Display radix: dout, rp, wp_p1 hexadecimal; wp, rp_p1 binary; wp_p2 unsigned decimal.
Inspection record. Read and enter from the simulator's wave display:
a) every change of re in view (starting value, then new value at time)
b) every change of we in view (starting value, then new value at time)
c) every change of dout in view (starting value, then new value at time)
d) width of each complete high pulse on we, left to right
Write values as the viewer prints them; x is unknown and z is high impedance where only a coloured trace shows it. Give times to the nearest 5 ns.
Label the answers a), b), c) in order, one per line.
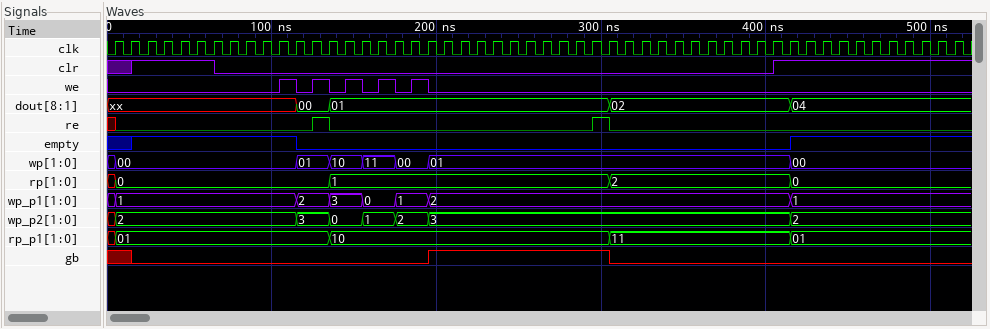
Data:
a) x, 0 at 5 ns, 1 at 125 ns, 0 at 135 ns, 1 at 295 ns, 0 at 305 ns
b) 0, 1 at 105 ns, 0 at 115 ns, 1 at 125 ns, 0 at 135 ns, 1 at 145 ns, 0 at 155 ns, 1 at 165 ns, 0 at 175 ns, 1 at 185 ns, 0 at 195 ns
c) xx, 00 at 115 ns, 01 at 135 ns, 02 at 305 ns, 04 at 415 ns
d) 10 ns, 10 ns, 10 ns, 10 ns, 10 ns
